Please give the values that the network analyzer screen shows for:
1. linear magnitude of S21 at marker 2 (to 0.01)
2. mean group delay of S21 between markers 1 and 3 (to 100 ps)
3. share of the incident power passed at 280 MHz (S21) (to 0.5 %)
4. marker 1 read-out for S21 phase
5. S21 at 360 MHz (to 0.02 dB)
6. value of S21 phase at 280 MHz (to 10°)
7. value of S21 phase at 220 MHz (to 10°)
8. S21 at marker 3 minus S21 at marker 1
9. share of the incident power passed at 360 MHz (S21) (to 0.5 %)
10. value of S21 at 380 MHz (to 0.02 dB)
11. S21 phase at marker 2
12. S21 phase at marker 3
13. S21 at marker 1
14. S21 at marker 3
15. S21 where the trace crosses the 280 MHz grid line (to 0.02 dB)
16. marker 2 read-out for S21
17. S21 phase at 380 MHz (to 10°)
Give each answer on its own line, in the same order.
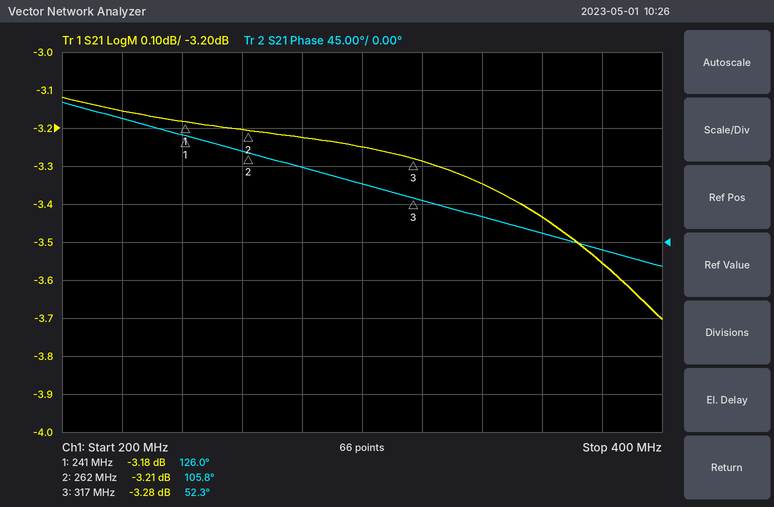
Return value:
0.69
2.7 ns
47.5 %
126.0°
-3.44 dB
90°
150°
-0.10 dB
45.5 %
-3.56 dB
105.8°
52.3°
-3.18 dB
-3.28 dB
-3.22 dB
-3.21 dB
-10°
